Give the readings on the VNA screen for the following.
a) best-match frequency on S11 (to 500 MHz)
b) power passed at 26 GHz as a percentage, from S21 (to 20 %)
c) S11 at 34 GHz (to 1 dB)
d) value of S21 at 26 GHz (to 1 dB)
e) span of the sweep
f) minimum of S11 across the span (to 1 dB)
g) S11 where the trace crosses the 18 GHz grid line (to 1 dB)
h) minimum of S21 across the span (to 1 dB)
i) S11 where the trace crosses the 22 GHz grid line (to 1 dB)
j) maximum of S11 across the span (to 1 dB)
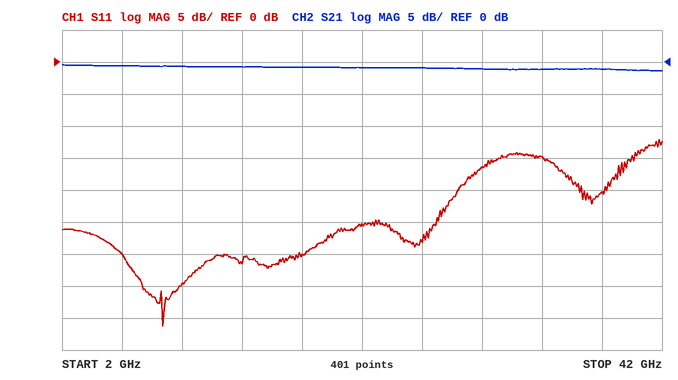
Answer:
8.5 GHz
80 %
-15 dB
-1 dB
40 GHz
-41 dB
-30 dB
-1 dB
-25 dB
-12 dB
